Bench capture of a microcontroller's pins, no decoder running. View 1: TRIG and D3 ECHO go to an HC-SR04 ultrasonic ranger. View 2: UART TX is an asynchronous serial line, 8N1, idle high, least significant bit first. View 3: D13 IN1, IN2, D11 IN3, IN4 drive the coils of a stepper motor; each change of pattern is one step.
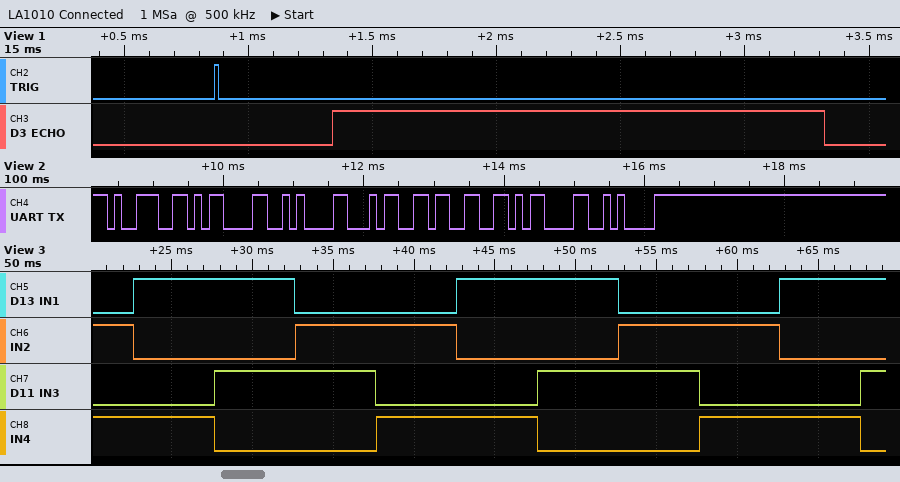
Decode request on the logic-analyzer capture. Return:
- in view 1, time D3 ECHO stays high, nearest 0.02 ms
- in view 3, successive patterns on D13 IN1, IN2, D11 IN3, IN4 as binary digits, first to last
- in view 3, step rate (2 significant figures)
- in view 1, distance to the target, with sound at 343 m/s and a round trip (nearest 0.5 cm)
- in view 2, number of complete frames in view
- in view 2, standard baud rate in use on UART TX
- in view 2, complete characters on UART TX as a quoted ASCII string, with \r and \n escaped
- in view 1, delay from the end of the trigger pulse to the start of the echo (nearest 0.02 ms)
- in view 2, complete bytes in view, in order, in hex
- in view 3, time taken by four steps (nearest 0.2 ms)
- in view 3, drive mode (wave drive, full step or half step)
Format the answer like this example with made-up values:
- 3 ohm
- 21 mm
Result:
- 1.98 ms
- 0101 1001 1010 0110 0101 1001 1010 0110 0101 1001 1010
- 200 steps/s
- 34 cm
- 7
- 9600 baud
- "9\r\n43\r\n"
- 0.46 ms
- 0x39 0x0D 0x0A 0x34 0x33 0x0D 0x0A
- 20.0 ms
- full step
